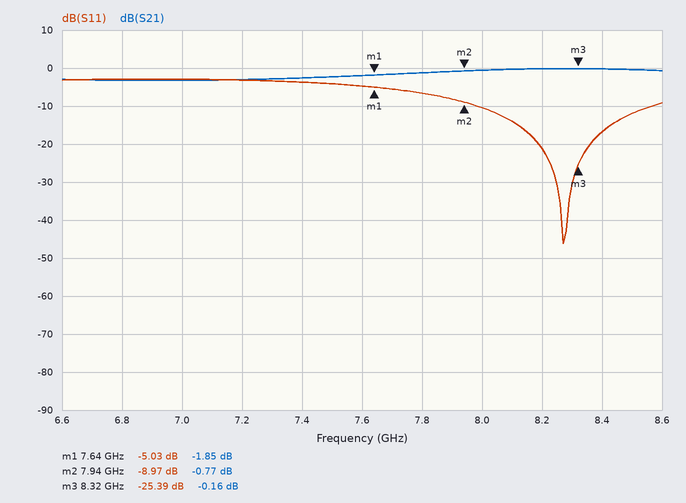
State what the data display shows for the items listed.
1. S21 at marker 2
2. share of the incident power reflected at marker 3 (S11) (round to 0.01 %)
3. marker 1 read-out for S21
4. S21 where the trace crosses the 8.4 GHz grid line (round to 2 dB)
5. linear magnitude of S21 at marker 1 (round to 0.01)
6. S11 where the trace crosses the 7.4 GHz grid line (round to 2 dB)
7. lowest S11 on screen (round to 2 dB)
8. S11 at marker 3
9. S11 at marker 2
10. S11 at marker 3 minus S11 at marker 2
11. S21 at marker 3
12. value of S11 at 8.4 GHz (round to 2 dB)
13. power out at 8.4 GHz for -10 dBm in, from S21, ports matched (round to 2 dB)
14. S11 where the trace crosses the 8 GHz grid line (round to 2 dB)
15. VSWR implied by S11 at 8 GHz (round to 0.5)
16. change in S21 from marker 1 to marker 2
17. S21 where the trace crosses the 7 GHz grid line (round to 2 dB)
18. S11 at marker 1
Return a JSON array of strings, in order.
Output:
["-0.77 dB", "0.29 %", "-1.85 dB", "0 dB", "0.81", "-4 dB", "-46 dB", "-25.39 dB", "-8.97 dB", "-16.42 dB", "-0.16 dB", "-16 dB", "-10 dBm", "-10 dB", "2.0", "1.08 dB", "-4 dB", "-5.03 dB"]
